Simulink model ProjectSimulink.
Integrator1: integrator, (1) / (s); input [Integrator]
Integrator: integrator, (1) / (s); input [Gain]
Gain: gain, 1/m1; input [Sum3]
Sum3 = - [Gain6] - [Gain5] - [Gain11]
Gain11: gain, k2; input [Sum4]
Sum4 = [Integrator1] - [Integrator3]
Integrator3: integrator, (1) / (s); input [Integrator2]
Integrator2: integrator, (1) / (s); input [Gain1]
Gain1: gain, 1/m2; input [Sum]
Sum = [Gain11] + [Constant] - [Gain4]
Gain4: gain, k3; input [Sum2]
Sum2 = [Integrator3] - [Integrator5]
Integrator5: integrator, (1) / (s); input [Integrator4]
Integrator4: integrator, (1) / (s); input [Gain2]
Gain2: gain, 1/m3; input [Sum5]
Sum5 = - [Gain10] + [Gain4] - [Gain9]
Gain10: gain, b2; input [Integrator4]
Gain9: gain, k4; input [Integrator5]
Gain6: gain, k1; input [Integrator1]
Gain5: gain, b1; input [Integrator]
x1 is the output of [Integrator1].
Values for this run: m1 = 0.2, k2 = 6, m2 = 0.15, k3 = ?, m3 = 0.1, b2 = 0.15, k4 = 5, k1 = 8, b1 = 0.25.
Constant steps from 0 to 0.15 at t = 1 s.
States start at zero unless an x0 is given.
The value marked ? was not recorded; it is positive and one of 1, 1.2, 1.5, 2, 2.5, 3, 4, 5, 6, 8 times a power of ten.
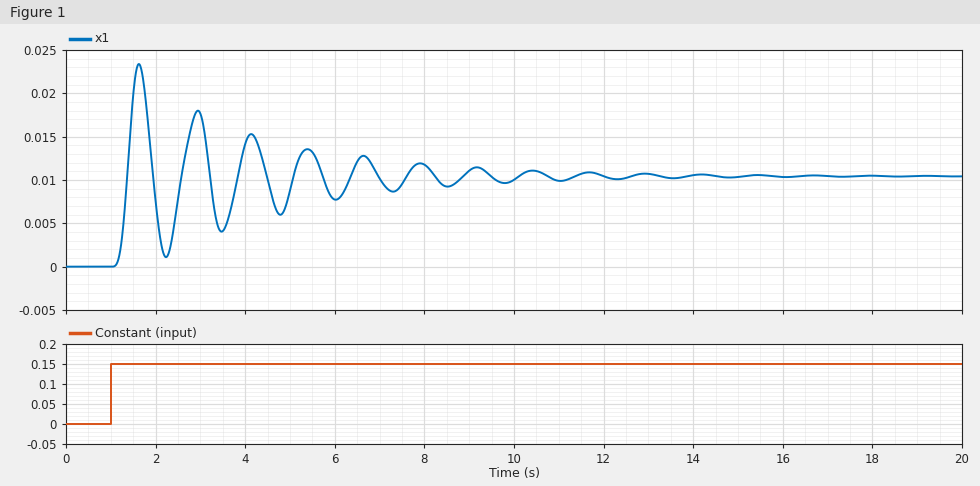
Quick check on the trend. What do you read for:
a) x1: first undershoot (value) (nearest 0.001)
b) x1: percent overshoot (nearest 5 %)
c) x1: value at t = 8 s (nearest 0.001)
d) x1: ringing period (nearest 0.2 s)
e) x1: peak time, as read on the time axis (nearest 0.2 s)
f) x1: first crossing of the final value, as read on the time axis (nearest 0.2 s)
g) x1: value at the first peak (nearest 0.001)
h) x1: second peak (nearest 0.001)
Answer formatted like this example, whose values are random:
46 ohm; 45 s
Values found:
0.001; 125 %; 0.012; 1.4 s; 1.6 s; 1.4 s; 0.023; 0.018
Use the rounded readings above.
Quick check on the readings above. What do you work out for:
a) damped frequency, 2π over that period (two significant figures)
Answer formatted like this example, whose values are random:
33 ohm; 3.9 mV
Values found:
4.5 rad/s
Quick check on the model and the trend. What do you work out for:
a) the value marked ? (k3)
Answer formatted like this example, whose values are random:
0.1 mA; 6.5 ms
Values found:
6
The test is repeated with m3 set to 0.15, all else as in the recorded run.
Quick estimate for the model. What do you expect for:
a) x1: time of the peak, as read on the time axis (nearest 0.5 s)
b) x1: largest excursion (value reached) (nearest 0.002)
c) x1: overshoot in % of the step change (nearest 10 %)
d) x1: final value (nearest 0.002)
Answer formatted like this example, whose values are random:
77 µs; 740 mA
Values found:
1.5 s; 0.022; 110 %; 0.010
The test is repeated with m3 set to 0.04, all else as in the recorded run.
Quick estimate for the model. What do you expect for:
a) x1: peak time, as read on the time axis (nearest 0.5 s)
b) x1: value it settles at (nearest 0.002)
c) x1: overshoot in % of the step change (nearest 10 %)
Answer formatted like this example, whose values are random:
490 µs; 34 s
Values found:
1.5 s; 0.010; 140 %
